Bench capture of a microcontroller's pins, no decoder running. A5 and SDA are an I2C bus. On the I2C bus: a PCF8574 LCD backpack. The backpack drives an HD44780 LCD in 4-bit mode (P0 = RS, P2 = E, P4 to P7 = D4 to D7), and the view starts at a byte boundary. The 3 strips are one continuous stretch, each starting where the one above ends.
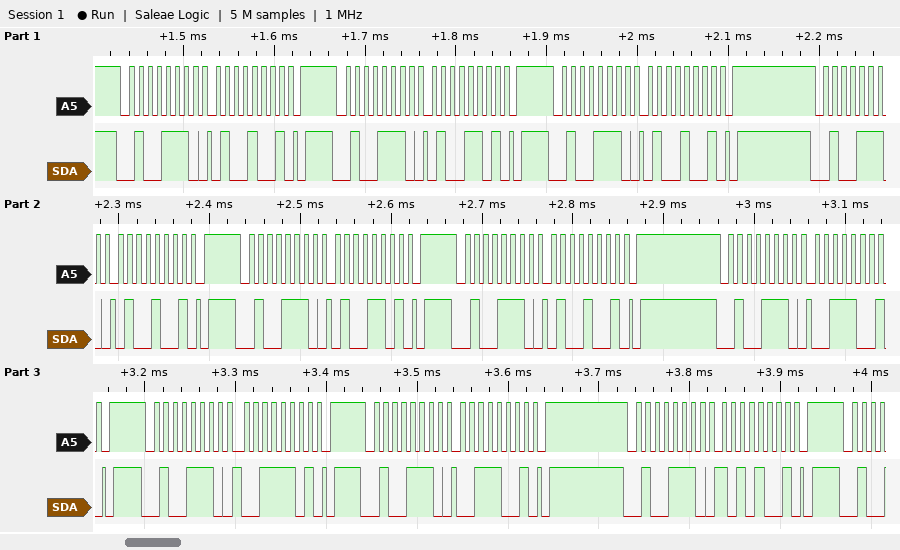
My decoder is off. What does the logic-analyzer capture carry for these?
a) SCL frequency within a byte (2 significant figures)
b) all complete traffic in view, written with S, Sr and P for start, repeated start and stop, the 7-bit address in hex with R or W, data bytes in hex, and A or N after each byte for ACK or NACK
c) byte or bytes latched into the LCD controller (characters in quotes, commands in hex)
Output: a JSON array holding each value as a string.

["100 kHz", "S 27W A 49 A P S 27W A 4D A P S 27W A 49 A P S 27W A 49 A P S 27W A 4D A P S 27W A 49 A P S 27W A 39 A P S 27W A 3D A P S 27W A 39 A P S 27W A A9 A P", "'D'"]
